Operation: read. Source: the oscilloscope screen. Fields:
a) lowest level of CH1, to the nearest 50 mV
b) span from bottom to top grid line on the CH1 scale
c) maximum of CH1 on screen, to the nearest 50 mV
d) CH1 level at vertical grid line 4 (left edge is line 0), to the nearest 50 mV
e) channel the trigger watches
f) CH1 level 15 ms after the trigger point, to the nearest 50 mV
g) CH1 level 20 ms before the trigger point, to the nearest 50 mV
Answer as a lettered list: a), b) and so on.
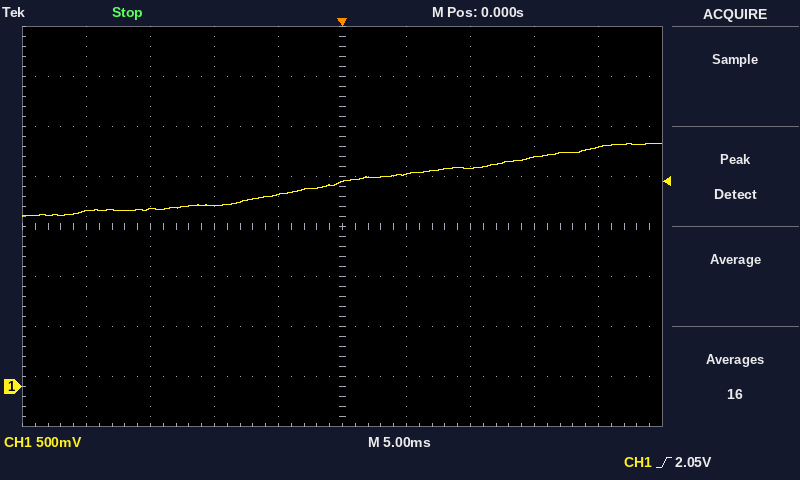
a) 1.70 V
b) 4 V
c) 2.45 V
d) 1.90 V
e) CH1
f) 2.30 V
g) 1.75 V
